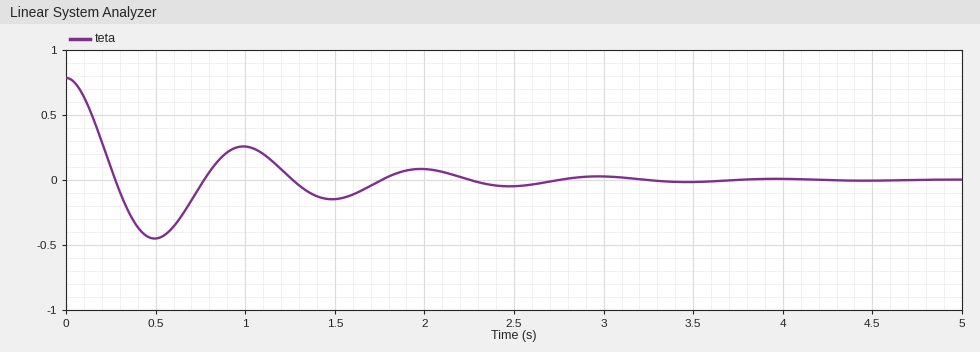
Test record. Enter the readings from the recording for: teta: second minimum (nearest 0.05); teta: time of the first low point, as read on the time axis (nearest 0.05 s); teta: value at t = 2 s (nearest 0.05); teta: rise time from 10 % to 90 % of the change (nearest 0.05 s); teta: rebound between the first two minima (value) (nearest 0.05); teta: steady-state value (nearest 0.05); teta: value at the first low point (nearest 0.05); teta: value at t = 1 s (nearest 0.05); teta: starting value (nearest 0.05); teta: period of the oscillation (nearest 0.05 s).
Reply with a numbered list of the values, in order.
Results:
1. -0.15
2. 0.50 s
3. 0.10
4. 0.20 s
5. 0.25
6. 0.00
7. -0.45
8. 0.25
9. 0.80
10. 1.00 s
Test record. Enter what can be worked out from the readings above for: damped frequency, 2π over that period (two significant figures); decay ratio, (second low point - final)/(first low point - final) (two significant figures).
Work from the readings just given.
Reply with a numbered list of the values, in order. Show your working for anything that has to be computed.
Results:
1. 2π / 1 = 6.3 rad/s
2. (-0.15 - 0) / (-0.45 - 0) = 0.33
